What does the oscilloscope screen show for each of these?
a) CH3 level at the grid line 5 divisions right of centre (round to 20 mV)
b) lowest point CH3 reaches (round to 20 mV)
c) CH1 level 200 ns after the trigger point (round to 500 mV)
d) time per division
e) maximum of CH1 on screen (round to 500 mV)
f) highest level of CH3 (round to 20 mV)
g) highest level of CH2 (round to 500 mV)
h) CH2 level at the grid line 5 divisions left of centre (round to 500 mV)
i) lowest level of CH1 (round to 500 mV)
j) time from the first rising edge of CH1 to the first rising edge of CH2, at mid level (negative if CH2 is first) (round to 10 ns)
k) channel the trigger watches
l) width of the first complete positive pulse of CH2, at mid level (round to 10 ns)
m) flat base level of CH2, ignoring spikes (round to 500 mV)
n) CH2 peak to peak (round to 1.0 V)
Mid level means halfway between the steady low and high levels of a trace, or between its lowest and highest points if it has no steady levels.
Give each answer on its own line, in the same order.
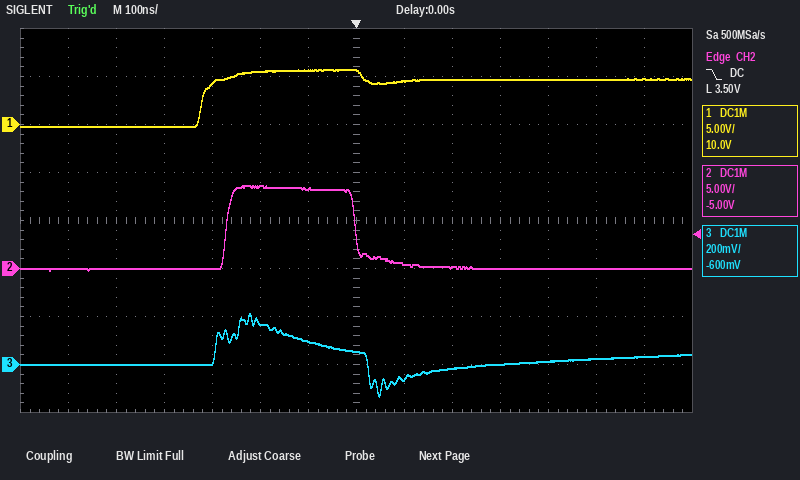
20 mV
-140 mV
4.5 V
100 ns
5.5 V
220 mV
8.5 V
0.0 V
0.0 V
+50 ns
CH2
270 ns
0.0 V
9.0 V
